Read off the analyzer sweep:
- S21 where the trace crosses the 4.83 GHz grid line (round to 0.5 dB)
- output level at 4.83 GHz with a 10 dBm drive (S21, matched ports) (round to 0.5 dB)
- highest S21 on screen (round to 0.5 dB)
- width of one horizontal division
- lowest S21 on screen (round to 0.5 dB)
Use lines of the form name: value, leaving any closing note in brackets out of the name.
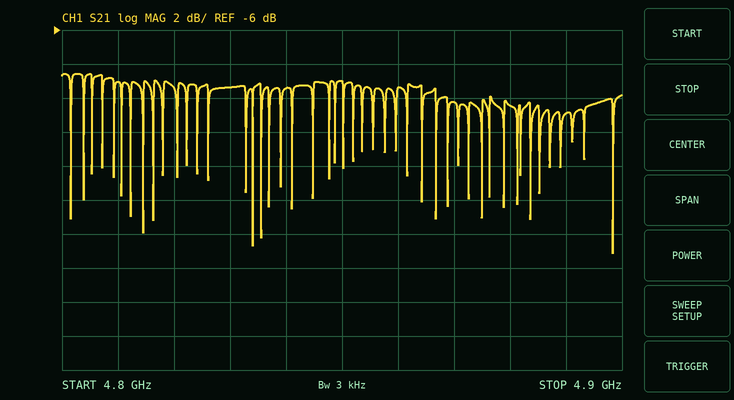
S21 where the trace crosses the 4.83 GHz grid line: -9.5 dB
output level at 4.83 GHz with a 10 dBm drive (S21, matched ports): 0.5 dBm
highest S21 on screen: -8.5 dB
width of one horizontal division: 10 MHz
lowest S21 on screen: -19.0 dB
